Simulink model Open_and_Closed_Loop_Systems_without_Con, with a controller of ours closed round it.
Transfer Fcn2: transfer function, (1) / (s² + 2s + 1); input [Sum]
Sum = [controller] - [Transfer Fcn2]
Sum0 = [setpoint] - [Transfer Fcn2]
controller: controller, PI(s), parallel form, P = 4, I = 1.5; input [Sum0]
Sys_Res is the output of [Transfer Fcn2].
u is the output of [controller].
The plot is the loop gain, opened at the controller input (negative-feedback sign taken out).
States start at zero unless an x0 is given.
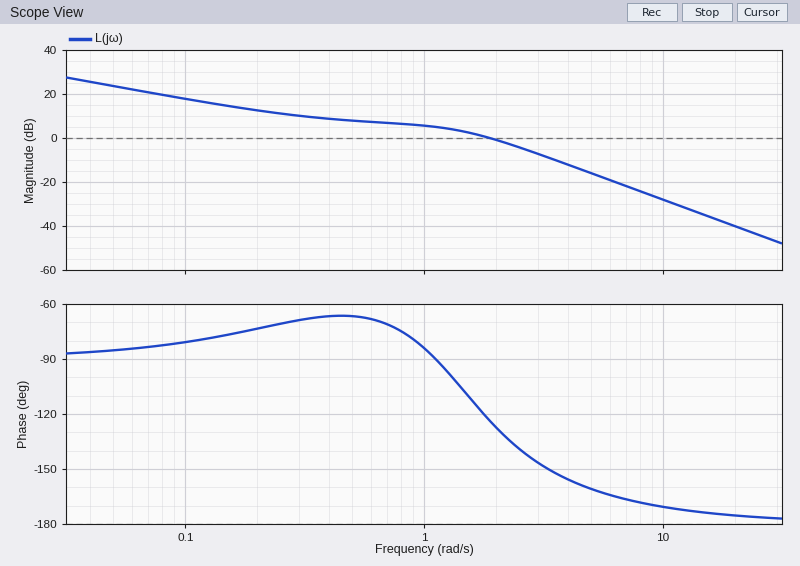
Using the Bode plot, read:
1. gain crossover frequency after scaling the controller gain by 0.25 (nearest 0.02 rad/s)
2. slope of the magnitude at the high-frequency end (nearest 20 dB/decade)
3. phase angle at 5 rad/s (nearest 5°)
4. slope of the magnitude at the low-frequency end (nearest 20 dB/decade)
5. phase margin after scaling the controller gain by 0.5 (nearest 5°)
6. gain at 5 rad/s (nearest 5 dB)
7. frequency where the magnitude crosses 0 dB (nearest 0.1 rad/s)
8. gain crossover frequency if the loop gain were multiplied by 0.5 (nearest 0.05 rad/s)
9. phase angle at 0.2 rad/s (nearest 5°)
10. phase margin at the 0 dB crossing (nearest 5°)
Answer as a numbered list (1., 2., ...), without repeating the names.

1. 0.22 rad/s
2. -40 dB/decade
3. -160°
4. -20 dB/decade
5. 100°
6. -15 dB
7. 1.9 rad/s
8. 0.90 rad/s
9. -75°
10. 55°
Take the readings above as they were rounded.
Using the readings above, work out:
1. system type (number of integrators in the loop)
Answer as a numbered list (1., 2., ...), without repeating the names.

1. 1
